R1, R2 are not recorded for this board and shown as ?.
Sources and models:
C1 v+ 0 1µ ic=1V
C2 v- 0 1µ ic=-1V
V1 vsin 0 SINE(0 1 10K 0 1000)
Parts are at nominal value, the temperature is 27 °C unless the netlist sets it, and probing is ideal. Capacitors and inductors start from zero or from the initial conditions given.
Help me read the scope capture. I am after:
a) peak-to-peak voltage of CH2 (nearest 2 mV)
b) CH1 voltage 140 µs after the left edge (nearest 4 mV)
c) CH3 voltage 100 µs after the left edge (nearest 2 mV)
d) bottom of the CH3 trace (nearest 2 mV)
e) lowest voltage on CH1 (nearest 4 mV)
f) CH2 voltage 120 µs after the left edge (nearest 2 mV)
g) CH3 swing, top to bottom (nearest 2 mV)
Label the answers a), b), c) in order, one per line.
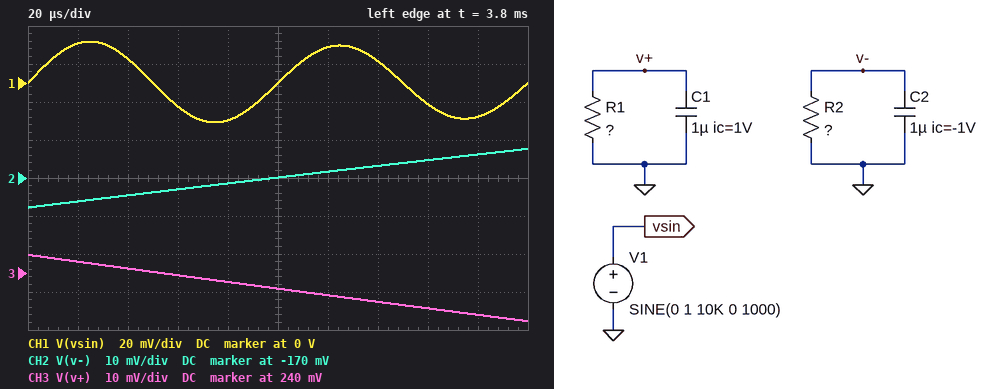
a) 16 mV
b) 12 mV
c) 236 mV
d) 228 mV
e) -20 mV
f) -168 mV
g) 18 mV
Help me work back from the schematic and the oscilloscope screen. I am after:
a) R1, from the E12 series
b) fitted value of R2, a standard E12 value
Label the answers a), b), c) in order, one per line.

a) 2.7 kΩ
b) 2.2 kΩ
